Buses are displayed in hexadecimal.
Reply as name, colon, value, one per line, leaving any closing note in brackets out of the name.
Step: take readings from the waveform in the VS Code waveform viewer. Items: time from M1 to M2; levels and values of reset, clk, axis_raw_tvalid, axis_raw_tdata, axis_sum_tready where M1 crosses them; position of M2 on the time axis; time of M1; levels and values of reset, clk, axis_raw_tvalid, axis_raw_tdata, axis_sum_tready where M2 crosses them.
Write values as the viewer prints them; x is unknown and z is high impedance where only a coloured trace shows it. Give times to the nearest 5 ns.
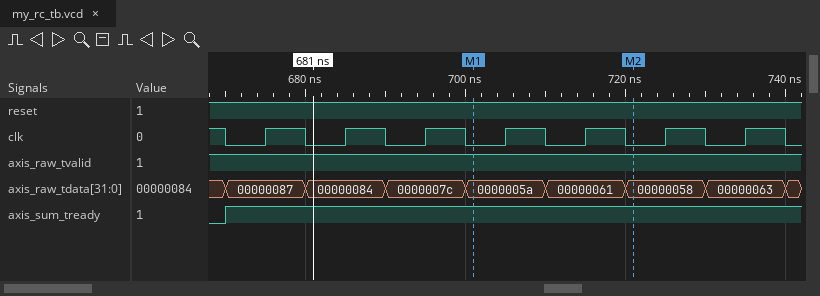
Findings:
time from M1 to M2: 20 ns
levels and values of reset, clk, axis_raw_tvalid, axis_raw_tdata, axis_sum_tready where M1 crosses them: reset=1, clk=0, axis_raw_tvalid=1, axis_raw_tdata=0000005a, axis_sum_tready=1
position of M2 on the time axis: 720 ns
time of M1: 700 ns
levels and values of reset, clk, axis_raw_tvalid, axis_raw_tdata, axis_sum_tready where M2 crosses them: reset=1, clk=0, axis_raw_tvalid=1, axis_raw_tdata=00000058, axis_sum_tready=1
